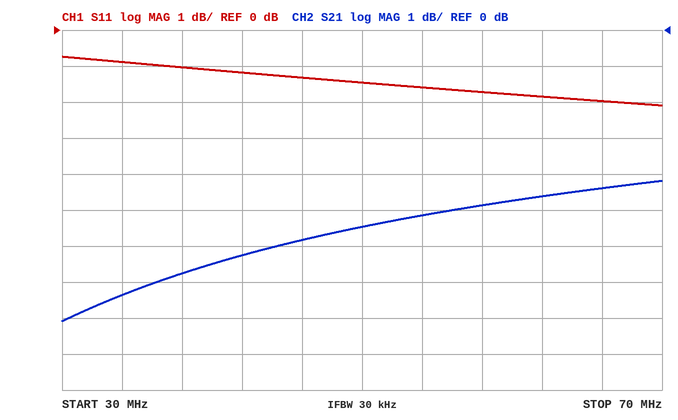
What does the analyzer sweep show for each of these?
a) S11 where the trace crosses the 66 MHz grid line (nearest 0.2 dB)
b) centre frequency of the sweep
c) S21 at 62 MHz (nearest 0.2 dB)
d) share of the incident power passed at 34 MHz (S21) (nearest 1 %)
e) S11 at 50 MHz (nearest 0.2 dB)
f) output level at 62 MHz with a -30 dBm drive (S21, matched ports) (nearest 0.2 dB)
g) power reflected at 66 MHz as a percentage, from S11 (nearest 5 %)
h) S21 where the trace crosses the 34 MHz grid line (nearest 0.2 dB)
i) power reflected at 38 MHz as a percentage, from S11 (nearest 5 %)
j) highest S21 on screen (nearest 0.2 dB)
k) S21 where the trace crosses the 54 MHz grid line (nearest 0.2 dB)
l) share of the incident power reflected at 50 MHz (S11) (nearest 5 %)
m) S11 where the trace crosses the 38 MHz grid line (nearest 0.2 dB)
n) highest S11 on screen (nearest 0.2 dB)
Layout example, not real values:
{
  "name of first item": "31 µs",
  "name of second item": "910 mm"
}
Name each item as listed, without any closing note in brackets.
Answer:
{
  "S11 where the trace crosses the 66 MHz grid line": "-2.0 dB",
  "centre frequency of the sweep": "50 MHz",
  "S21 at 62 MHz": "-4.6 dB",
  "share of the incident power passed at 34 MHz (S21)": "18 %",
  "S11 at 50 MHz": "-1.4 dB",
  "output level at 62 MHz with a -30 dBm drive (S21, matched ports)": "-34.6 dBm",
  "power reflected at 66 MHz as a percentage, from S11": "65 %",
  "S21 where the trace crosses the 34 MHz grid line": "-7.4 dB",
  "power reflected at 38 MHz as a percentage, from S11": "80 %",
  "highest S21 on screen": "-4.2 dB",
  "S21 where the trace crosses the 54 MHz grid line": "-5.2 dB",
  "share of the incident power reflected at 50 MHz (S11)": "70 %",
  "S11 where the trace crosses the 38 MHz grid line": "-1.0 dB",
  "highest S11 on screen": "-0.8 dB"
}
